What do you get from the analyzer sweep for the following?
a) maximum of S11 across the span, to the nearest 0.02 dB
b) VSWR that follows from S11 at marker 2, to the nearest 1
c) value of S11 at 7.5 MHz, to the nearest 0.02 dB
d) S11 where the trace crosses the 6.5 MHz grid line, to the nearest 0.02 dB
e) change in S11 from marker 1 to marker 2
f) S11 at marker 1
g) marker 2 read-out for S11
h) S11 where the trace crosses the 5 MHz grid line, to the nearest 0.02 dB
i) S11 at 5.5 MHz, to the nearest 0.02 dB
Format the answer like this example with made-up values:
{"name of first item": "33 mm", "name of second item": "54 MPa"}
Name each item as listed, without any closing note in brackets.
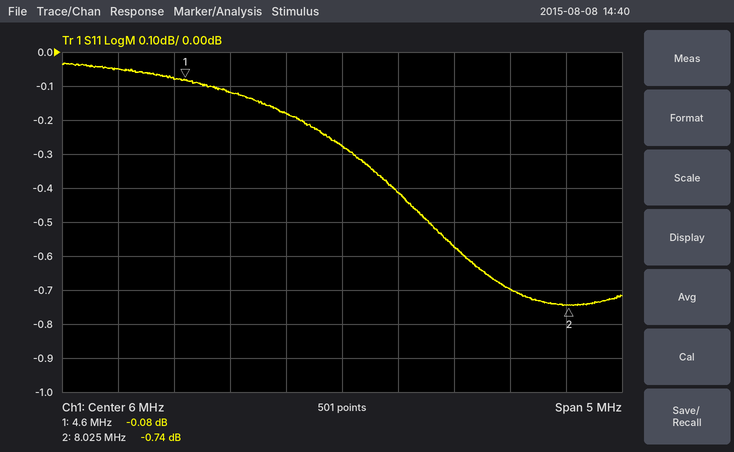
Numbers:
{"maximum of S11 across the span, to the nearest 0.02 dB": "-0.04 dB", "VSWR that follows from S11 at marker 2, to the nearest 1": "23", "value of S11 at 7.5 MHz, to the nearest 0.02 dB": "-0.70 dB", "S11 where the trace crosses the 6.5 MHz grid line, to the nearest 0.02 dB": "-0.42 dB", "change in S11 from marker 1 to marker 2": "-0.66 dB", "S11 at marker 1": "-0.08 dB", "marker 2 read-out for S11": "-0.74 dB", "S11 where the trace crosses the 5 MHz grid line, to the nearest 0.02 dB": "-0.12 dB", "S11 at 5.5 MHz, to the nearest 0.02 dB": "-0.18 dB"}
